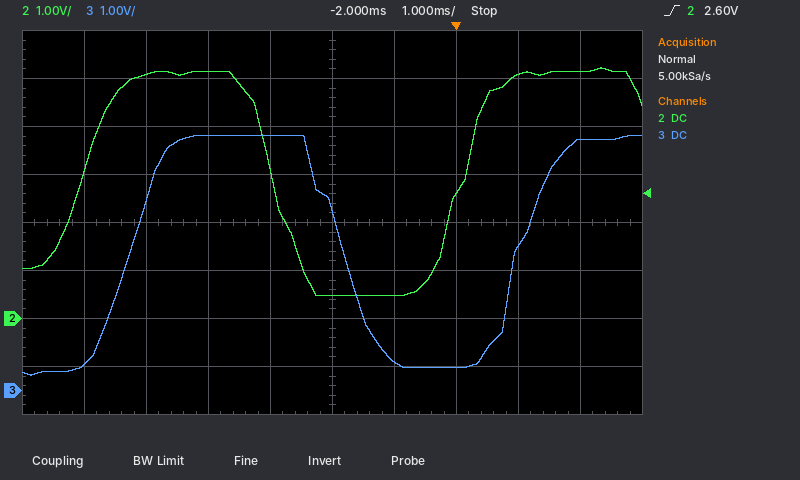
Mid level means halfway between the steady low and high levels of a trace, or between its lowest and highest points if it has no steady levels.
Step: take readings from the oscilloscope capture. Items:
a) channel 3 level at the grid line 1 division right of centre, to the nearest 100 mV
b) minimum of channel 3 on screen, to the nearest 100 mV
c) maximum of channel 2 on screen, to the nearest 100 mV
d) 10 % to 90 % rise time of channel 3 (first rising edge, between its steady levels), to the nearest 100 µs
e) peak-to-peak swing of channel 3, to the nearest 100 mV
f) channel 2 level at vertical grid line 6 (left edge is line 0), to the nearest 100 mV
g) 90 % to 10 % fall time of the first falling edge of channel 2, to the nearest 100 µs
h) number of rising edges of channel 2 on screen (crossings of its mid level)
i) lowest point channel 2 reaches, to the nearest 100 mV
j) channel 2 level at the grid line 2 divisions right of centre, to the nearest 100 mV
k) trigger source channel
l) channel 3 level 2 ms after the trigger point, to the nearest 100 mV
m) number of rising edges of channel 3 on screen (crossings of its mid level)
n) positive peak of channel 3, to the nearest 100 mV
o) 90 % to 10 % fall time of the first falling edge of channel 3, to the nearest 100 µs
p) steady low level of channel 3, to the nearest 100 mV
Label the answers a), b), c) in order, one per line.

a) 600 mV
b) 300 mV
c) 5.2 V
d) 1.0 ms
e) 5.0 V
f) 500 mV
g) 900 µs
h) 2
i) 500 mV
j) 2.6 V
k) channel 2
l) 5.2 V
m) 2
n) 5.3 V
o) 1.1 ms
p) 500 mV
